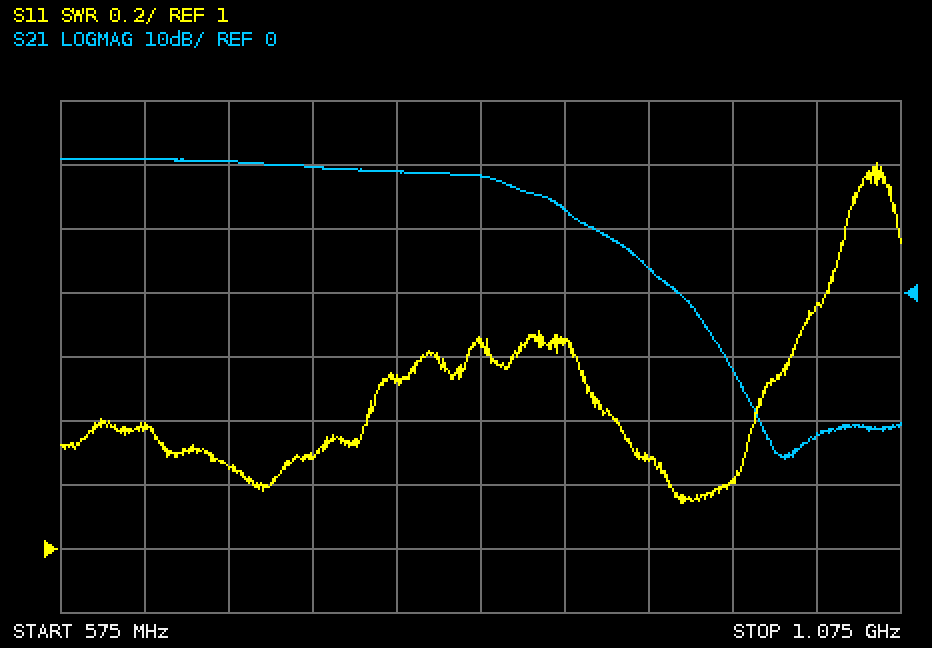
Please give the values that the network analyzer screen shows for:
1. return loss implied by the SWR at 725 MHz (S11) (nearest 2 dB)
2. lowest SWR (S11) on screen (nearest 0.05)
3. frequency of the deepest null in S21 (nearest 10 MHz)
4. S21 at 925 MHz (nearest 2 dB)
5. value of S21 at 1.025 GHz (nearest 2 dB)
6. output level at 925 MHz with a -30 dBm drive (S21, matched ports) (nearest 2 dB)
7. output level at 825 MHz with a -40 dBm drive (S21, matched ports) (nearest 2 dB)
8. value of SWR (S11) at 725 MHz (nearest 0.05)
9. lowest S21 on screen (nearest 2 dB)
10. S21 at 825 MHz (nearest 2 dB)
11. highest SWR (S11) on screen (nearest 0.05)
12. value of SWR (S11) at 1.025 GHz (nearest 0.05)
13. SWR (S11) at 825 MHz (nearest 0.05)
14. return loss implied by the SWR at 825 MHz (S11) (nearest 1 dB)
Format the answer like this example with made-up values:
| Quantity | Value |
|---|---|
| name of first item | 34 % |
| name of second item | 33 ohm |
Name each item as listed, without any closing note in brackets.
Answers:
| Quantity | Value |
|---|---|
| return loss implied by the SWR at 725 MHz (S11) | 18 dB |
| lowest SWR (S11) on screen | 1.15 |
| frequency of the deepest null in S21 | 1.01 GHz |
| S21 at 925 MHz | 4 dB |
| value of S21 at 1.025 GHz | -22 dB |
| output level at 925 MHz with a -30 dBm drive (S21, matched ports) | -26 dBm |
| output level at 825 MHz with a -40 dBm drive (S21, matched ports) | -22 dBm |
| value of SWR (S11) at 725 MHz | 1.30 |
| lowest S21 on screen | -26 dB |
| S21 at 825 MHz | 18 dB |
| highest SWR (S11) on screen | 2.20 |
| value of SWR (S11) at 1.025 GHz | 1.75 |
| SWR (S11) at 825 MHz | 1.65 |
| return loss implied by the SWR at 825 MHz (S11) | 12 dB |
